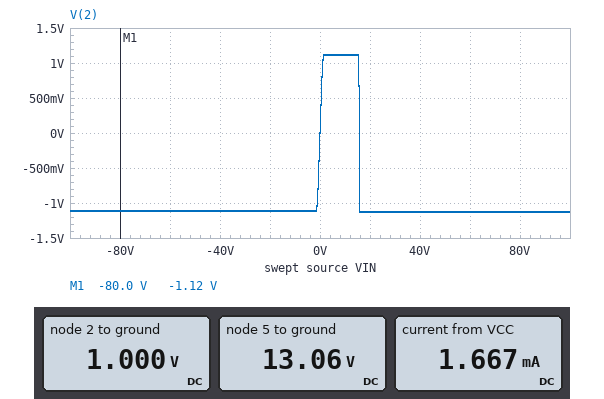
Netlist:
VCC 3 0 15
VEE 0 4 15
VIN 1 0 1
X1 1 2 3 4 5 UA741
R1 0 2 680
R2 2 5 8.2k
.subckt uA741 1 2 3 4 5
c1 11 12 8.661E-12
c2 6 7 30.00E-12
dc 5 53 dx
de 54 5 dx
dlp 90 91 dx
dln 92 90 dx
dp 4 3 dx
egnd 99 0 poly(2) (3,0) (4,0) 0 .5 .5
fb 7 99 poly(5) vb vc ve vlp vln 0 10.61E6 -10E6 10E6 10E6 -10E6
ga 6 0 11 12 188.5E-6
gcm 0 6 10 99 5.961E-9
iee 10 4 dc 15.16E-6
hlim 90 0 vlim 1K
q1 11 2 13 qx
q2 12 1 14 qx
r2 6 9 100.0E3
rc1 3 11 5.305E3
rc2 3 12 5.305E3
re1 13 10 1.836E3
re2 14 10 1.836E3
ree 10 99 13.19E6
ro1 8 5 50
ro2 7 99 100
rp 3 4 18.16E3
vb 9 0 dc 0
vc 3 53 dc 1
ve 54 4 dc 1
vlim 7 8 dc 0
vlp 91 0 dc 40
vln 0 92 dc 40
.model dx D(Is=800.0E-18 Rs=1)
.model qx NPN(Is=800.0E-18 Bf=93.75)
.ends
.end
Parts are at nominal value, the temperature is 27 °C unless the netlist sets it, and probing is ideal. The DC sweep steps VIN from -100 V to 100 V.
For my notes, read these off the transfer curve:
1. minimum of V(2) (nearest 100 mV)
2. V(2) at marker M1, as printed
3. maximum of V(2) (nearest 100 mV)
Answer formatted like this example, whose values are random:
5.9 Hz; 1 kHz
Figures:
-1.1 V; -1.12 V; 1.1 V
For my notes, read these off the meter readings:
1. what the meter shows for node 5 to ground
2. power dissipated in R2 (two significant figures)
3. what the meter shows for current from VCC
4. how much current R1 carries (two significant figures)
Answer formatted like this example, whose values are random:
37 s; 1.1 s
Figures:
13.06 V; 18 mW; 1.667 mA; 1.5 mA
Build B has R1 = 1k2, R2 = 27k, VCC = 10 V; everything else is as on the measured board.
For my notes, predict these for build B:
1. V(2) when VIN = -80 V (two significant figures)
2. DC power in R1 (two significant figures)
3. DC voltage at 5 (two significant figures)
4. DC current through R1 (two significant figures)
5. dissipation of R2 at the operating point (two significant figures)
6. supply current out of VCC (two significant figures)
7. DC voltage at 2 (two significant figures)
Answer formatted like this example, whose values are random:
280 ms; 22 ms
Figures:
-620 mV; 140 µW; 9.6 V; 340 µA; 3.1 mW; 1.4 mA; 410 mV
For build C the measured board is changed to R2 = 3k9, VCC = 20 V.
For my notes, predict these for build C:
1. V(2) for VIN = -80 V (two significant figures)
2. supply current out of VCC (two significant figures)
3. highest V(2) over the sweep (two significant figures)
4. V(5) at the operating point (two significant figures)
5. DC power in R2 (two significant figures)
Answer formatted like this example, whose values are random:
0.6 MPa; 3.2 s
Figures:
-2.2 V; 1.9 mA; 2.9 V; 6.7 V; 8.4 mW
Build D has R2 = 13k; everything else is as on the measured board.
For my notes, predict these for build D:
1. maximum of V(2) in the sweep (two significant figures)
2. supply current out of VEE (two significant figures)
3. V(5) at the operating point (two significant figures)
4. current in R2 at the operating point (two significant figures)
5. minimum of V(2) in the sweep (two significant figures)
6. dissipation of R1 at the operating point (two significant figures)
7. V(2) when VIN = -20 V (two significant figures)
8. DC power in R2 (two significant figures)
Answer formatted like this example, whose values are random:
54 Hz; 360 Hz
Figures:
730 mV; 1.7 mA; 15 V; 1.1 mA; -740 mV; 780 µW; -730 mV; 15 mW
